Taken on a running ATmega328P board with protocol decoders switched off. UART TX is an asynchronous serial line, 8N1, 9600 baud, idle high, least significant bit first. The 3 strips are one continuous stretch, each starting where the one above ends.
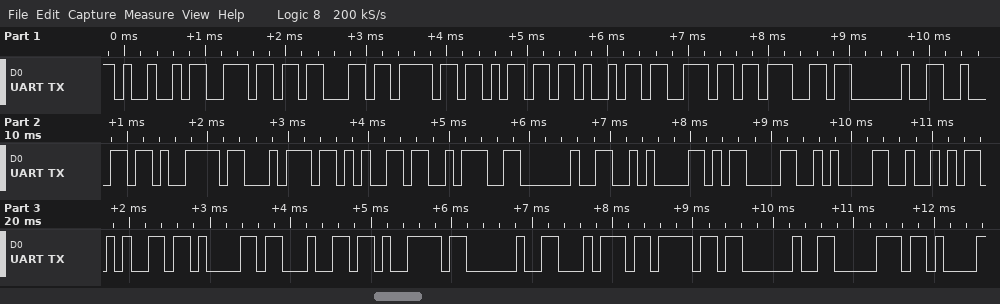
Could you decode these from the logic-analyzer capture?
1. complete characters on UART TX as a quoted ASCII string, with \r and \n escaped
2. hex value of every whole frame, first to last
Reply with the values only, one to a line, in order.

"Incoming byte: \n\r\nReady to p"
49 6E 63 6F 6D 69 6E 67 20 62 79 74 65 3A 20 0A 0D 0A 52 65 61 64 79 20 74 6F 20 70
